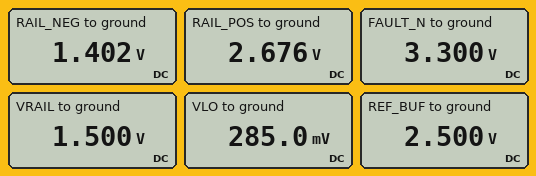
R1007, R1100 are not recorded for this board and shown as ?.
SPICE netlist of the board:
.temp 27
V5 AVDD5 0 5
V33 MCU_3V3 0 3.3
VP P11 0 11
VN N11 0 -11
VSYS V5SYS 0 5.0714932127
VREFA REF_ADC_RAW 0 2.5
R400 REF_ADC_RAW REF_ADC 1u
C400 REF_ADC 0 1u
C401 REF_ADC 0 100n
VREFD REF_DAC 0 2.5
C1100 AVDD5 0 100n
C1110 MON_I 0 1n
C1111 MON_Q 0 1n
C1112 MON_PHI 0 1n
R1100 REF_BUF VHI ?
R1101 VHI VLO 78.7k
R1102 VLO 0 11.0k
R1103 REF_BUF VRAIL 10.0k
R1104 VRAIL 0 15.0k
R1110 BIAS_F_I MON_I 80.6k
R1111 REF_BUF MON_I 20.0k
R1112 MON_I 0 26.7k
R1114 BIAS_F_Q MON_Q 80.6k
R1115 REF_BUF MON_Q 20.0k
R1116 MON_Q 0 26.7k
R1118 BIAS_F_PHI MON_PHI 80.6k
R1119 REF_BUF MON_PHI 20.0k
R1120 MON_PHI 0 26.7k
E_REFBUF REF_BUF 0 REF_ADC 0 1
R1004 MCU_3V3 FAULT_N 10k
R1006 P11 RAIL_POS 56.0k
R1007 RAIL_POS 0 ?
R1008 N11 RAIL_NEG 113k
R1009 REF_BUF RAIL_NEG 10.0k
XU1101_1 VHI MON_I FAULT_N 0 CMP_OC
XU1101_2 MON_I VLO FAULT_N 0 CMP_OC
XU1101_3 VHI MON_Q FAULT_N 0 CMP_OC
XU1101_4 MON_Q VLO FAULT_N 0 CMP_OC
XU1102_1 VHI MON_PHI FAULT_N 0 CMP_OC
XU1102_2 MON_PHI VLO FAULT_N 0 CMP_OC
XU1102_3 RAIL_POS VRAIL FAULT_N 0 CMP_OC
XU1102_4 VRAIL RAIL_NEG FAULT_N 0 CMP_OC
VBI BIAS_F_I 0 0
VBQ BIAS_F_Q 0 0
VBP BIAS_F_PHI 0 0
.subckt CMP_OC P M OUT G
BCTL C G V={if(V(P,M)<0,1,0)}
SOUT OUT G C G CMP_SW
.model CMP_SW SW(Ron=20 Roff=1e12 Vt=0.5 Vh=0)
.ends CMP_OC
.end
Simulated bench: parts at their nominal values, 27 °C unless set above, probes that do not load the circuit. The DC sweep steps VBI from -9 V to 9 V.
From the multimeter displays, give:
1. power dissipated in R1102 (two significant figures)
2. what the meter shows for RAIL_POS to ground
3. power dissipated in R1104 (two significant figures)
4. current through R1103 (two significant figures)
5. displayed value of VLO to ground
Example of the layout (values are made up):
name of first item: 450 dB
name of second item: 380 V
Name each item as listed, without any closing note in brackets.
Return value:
power dissipated in R1102: 7.4 µW
what the meter shows for RAIL_POS to ground: 2.676 V
power dissipated in R1104: 150 µW
current through R1103: 100 µA
displayed value of VLO to ground: 285.0 mV
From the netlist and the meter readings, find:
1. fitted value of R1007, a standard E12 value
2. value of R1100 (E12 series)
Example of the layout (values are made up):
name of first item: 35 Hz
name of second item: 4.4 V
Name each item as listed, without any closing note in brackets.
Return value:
fitted value of R1007, a standard E12 value: 18 kΩ
value of R1100: 6.8 kΩ
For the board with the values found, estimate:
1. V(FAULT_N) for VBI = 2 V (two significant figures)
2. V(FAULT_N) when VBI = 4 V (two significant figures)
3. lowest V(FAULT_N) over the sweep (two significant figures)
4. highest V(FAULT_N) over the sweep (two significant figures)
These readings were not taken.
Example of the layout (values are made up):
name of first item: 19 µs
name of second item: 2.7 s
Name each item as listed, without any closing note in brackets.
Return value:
V(FAULT_N) for VBI = 2 V: 3.3 V
V(FAULT_N) when VBI = 4 V: 3.3 V
lowest V(FAULT_N) over the sweep: 6.6 mV
highest V(FAULT_N) over the sweep: 3.3 V
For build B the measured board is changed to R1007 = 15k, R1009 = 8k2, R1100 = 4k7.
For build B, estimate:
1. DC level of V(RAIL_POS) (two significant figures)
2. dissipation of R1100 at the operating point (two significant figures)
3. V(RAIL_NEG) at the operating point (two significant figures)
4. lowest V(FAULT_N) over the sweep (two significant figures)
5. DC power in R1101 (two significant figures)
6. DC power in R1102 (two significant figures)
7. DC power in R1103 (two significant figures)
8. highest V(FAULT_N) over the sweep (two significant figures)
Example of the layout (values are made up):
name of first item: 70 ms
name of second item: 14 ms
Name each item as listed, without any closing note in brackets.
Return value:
DC level of V(RAIL_POS): 2.3 V
dissipation of R1100 at the operating point: 3.3 µW
V(RAIL_NEG) at the operating point: 1.6 V
lowest V(FAULT_N) over the sweep: 3.3 mV
DC power in R1101: 55 µW
DC power in R1102: 7.7 µW
DC power in R1103: 100 µW
highest V(FAULT_N) over the sweep: 6.6 mV
